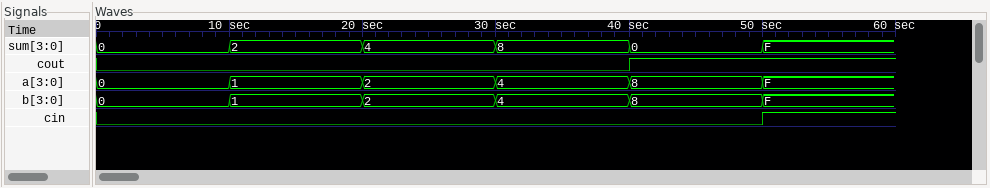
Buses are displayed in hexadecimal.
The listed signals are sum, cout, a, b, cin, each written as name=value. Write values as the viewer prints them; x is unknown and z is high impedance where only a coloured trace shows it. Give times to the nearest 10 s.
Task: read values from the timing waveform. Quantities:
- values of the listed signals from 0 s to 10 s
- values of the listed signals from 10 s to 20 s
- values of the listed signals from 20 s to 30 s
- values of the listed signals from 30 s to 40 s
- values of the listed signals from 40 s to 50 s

sum=0, cout=0, a=0, b=0, cin=0
sum=2, cout=0, a=1, b=1, cin=0
sum=4, cout=0, a=2, b=2, cin=0
sum=8, cout=0, a=4, b=4, cin=0
sum=0, cout=1, a=8, b=8, cin=0
